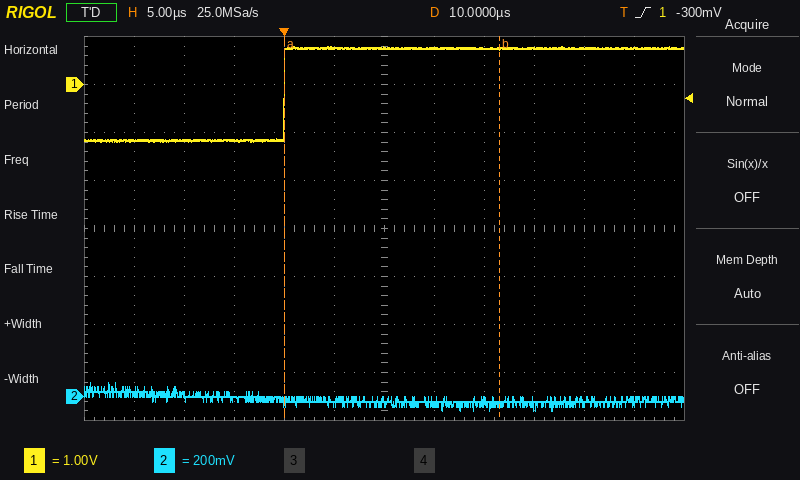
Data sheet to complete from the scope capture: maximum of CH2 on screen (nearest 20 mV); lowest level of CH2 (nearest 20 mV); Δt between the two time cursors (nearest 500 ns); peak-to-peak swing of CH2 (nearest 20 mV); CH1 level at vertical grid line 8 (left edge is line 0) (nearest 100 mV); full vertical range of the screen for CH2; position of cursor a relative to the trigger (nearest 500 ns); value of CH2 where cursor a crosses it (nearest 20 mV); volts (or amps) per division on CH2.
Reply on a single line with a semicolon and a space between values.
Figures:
60 mV; -60 mV; 21.5 µs; 120 mV; 800 mV; 1.6 V; 0.0 µs; -20 mV; 200 mV
